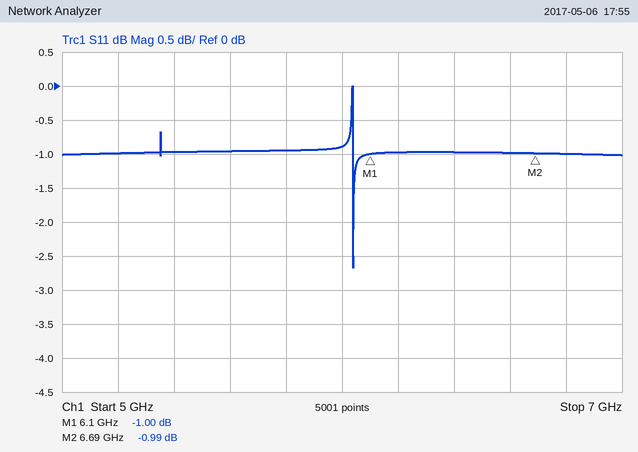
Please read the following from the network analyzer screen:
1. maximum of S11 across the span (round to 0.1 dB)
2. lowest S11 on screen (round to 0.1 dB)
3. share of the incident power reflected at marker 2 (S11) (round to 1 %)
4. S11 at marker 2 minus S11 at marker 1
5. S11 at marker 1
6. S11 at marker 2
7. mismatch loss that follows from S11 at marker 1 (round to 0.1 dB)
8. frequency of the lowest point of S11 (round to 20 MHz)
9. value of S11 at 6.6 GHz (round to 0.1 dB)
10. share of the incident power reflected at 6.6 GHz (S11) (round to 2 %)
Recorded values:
0.0 dB
-2.7 dB
80 %
0.01 dB
-1.00 dB
-0.99 dB
6.9 dB
6.04 GHz
-1.0 dB
80 %
